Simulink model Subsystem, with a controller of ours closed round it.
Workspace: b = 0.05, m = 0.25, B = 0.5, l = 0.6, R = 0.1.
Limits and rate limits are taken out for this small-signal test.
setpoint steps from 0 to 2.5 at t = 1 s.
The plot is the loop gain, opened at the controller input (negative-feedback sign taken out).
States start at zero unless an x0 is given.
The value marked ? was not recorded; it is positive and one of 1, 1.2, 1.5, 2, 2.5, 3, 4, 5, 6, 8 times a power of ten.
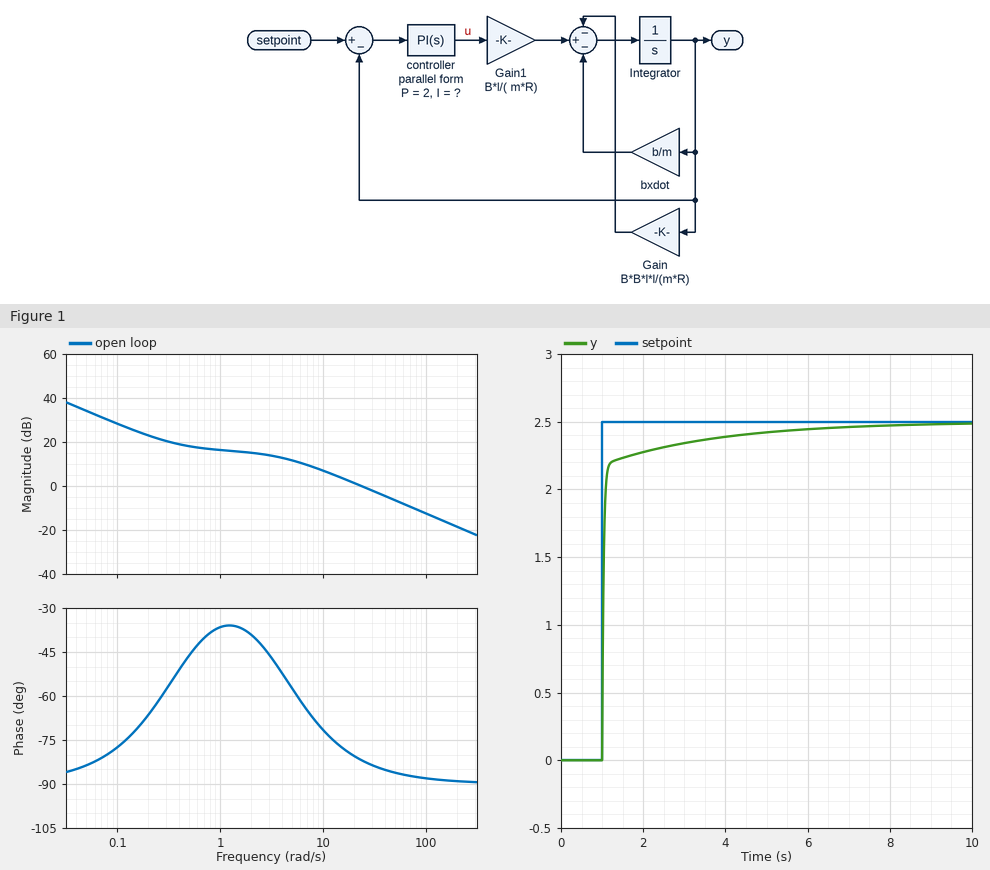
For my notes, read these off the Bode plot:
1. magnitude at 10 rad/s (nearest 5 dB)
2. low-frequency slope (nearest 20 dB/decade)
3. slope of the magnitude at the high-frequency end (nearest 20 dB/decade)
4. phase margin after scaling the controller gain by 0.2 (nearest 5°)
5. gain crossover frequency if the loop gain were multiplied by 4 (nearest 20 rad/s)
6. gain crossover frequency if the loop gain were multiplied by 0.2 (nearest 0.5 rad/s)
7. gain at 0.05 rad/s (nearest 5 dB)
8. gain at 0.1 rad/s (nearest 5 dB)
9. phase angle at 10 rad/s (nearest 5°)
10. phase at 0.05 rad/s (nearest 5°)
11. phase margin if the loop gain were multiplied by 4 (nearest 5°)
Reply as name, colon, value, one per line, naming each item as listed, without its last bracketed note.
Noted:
magnitude at 10 rad/s: 5 dB
low-frequency slope: -20 dB/decade
slope of the magnitude at the high-frequency end: -20 dB/decade
phase margin after scaling the controller gain by 0.2: 135°
gain crossover frequency if the loop gain were multiplied by 4: 100 rad/s
gain crossover frequency if the loop gain were multiplied by 0.2: 3.0 rad/s
gain at 0.05 rad/s: 35 dB
gain at 0.1 rad/s: 30 dB
phase angle at 10 rad/s: -70°
phase at 0.05 rad/s: -85°
phase margin if the loop gain were multiplied by 4: 90°
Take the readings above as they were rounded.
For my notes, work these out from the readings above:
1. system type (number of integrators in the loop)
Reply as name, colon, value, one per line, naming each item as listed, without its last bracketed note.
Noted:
system type: 1
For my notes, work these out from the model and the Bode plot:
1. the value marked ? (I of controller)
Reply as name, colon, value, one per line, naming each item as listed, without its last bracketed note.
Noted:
the value marked ?: 0.8
